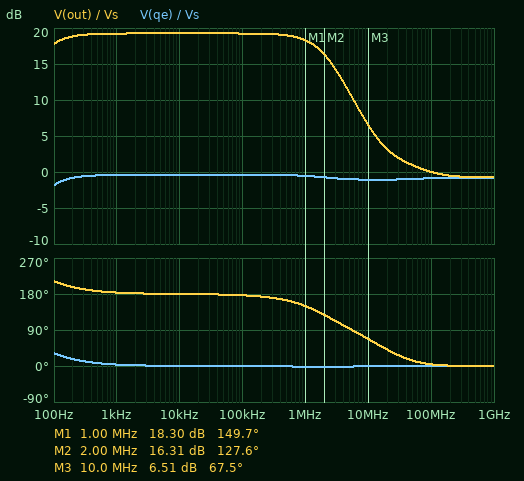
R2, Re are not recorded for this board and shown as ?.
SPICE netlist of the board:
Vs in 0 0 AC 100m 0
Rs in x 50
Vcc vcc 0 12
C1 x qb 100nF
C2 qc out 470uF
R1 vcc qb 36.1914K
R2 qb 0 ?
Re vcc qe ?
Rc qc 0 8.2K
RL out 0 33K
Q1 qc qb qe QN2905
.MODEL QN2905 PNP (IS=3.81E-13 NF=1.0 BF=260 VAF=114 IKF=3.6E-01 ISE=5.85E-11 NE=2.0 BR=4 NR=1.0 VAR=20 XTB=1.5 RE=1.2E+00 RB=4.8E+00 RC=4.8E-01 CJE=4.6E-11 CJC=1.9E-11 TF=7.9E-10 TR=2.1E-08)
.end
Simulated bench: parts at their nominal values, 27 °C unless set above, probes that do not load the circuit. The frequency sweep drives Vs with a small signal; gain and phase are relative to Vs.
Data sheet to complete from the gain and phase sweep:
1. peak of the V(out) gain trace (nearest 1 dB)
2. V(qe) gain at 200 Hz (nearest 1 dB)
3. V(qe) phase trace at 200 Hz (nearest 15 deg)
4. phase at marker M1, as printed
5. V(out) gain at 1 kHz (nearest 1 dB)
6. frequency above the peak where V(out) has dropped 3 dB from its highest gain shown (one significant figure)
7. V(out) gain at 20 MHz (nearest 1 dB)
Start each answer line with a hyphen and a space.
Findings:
- 19 dB
- -1 dB
- 15 deg
- 149.7 deg
- 19 dB
- 2 MHz
- 3 dB
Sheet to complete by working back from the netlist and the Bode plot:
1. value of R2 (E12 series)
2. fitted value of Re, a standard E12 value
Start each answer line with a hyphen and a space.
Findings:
- 270 kΩ
- 680 Ω
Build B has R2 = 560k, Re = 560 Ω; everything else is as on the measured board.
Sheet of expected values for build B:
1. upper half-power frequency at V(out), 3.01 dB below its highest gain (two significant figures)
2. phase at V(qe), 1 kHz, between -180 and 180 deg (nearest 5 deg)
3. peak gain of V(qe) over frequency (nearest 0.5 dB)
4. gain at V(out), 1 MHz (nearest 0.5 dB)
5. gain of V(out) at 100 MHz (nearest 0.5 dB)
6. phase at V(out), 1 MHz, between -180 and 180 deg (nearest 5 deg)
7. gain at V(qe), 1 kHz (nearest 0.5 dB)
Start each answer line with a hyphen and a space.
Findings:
- 2.8 MHz
- 5 deg
- -1.0 dB
- 19.0 dB
- -0.5 dB
- 155 deg
- -1.5 dB
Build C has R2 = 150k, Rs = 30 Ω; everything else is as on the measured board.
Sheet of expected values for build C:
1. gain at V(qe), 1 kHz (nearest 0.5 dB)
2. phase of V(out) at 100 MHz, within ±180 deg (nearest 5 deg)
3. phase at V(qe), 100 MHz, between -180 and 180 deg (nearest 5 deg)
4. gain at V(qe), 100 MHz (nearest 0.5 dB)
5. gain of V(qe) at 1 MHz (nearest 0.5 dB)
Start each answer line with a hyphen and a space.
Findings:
- -8.0 dB
- 0 deg
- 0 deg
- -0.5 dB
- -1.0 dB
